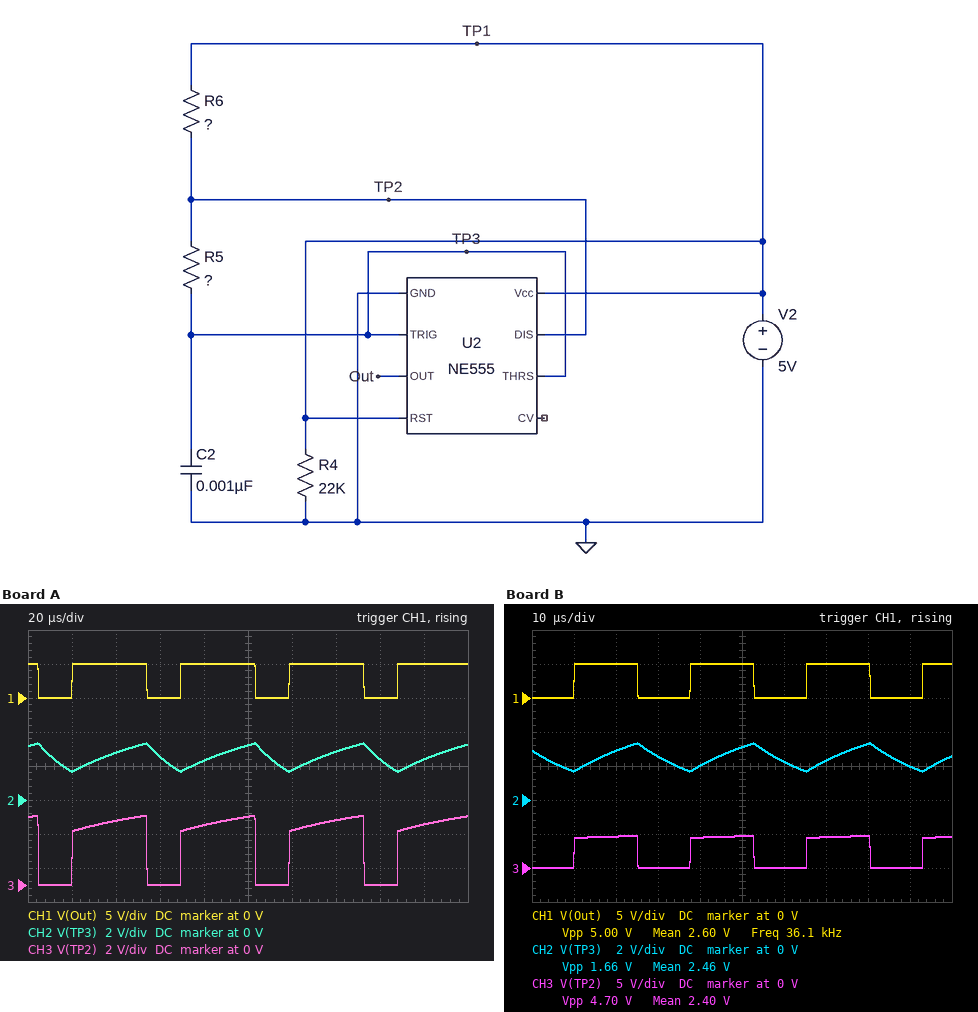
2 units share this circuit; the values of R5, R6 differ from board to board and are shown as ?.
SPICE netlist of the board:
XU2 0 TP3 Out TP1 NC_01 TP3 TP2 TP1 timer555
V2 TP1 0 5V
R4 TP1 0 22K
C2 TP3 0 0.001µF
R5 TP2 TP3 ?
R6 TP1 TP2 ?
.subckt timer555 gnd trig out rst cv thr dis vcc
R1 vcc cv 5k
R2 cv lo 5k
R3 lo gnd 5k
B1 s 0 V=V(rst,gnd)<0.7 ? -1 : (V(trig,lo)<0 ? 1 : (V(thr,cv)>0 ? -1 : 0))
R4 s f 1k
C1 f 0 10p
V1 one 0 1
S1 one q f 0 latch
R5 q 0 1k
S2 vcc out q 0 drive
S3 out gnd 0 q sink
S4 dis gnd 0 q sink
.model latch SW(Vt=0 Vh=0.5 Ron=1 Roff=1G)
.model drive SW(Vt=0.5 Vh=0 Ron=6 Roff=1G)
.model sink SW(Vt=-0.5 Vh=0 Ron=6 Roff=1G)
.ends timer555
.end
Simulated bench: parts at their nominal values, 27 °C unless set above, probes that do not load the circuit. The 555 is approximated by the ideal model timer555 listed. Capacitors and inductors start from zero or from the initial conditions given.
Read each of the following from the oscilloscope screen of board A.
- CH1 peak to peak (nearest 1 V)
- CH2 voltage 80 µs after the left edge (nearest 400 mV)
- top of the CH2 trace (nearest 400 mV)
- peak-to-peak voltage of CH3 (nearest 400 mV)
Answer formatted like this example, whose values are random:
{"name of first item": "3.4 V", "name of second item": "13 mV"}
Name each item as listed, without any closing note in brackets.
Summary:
{"CH1 peak to peak": "5 V", "CH2 voltage 80 µs after the left edge": "2.4 V", "top of the CH2 trace": "3.2 V", "peak-to-peak voltage of CH3": "4.0 V"}
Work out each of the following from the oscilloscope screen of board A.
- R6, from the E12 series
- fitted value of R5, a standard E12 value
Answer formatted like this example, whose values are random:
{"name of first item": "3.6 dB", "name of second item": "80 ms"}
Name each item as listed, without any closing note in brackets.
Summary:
{"R6, from the E12 series": "27 kΩ", "fitted value of R5, a standard E12 value": "22 kΩ"}
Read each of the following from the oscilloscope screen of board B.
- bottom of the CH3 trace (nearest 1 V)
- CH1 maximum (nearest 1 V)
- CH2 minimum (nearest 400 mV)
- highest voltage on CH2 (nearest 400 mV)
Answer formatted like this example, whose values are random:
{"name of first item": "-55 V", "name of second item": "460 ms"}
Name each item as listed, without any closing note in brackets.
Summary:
{"bottom of the CH3 trace": "0 V", "CH1 maximum": "5 V", "CH2 minimum": "1.6 V", "highest voltage on CH2": "3.2 V"}
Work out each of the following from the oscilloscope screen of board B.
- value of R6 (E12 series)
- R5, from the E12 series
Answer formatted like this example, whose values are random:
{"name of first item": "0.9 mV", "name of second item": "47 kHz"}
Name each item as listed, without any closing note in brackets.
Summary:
{"value of R6": "3.9 kΩ", "R5, from the E12 series": "18 kΩ"}
